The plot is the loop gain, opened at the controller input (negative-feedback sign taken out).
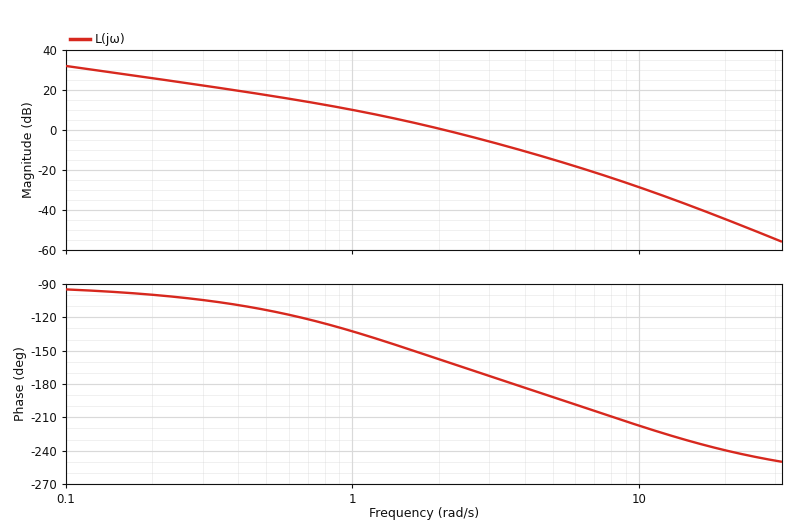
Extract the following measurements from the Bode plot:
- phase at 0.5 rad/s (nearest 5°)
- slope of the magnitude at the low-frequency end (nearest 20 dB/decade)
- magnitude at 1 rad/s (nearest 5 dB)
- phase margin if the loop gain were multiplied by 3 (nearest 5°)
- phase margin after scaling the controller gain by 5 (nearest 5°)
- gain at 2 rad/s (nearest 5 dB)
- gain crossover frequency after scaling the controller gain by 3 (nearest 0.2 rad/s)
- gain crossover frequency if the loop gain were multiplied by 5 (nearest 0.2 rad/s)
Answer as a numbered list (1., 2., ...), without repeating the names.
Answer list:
1. -115°
2. -20 dB/decade
3. 10 dB
4. 0°
5. -10°
6. 0 dB
7. 3.8 rad/s
8. 4.8 rad/s
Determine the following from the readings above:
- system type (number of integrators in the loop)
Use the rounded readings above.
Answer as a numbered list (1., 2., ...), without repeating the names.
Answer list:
1. 1
